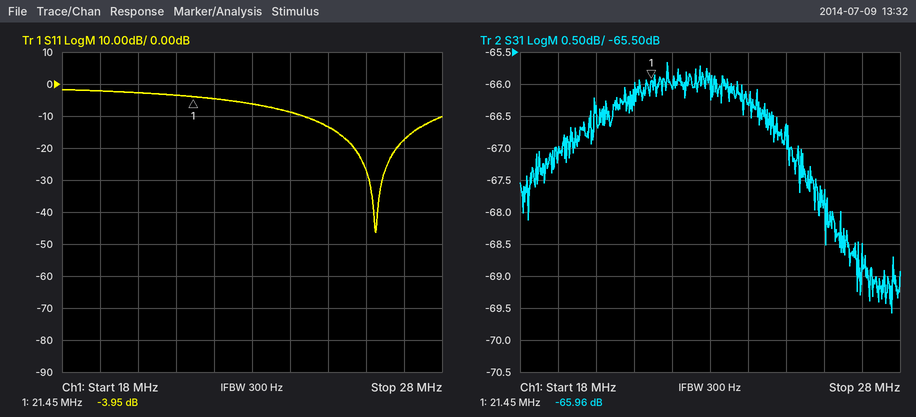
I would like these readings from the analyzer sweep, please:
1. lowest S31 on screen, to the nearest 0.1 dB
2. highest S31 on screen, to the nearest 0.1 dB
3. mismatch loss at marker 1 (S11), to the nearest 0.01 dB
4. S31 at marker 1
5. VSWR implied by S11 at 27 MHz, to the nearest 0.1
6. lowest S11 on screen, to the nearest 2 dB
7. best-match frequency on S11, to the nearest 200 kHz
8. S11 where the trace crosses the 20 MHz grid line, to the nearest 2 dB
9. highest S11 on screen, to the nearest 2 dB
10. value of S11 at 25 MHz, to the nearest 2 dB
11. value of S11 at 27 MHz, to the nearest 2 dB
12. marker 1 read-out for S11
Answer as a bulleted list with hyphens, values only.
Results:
- -69.6 dB
- -65.7 dB
- 2.24 dB
- -65.96 dB
- 1.3
- -46 dB
- 26.2 MHz
- -2 dB
- -2 dB
- -14 dB
- -18 dB
- -3.95 dB
